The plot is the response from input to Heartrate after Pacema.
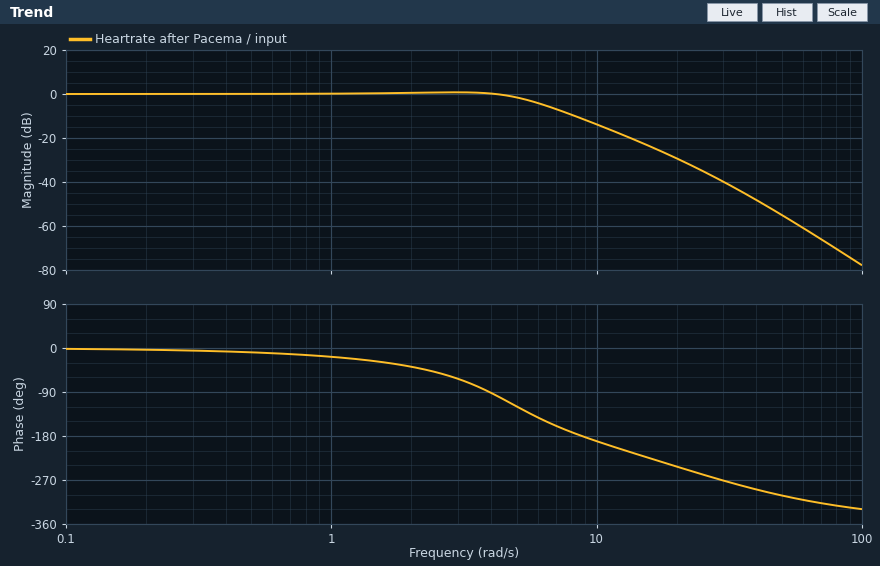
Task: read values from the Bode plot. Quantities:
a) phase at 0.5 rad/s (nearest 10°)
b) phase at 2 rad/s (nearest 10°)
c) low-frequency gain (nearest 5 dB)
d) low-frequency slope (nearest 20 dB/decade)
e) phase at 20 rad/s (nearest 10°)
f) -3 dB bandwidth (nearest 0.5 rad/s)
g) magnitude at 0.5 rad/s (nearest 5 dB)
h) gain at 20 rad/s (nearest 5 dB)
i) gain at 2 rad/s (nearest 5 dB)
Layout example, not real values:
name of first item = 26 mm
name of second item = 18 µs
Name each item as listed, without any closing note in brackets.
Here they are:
phase at 0.5 rad/s = -10°
phase at 2 rad/s = -40°
low-frequency gain = 0 dB
low-frequency slope = 0 dB/decade
phase at 20 rad/s = -240°
-3 dB bandwidth = 5.5 rad/s
magnitude at 0.5 rad/s = 0 dB
gain at 20 rad/s = -30 dB
gain at 2 rad/s = 0 dB
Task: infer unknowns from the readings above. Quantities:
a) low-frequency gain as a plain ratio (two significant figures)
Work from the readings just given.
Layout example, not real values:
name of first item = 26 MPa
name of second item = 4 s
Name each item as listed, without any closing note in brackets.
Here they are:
low-frequency gain as a plain ratio = 1.0
